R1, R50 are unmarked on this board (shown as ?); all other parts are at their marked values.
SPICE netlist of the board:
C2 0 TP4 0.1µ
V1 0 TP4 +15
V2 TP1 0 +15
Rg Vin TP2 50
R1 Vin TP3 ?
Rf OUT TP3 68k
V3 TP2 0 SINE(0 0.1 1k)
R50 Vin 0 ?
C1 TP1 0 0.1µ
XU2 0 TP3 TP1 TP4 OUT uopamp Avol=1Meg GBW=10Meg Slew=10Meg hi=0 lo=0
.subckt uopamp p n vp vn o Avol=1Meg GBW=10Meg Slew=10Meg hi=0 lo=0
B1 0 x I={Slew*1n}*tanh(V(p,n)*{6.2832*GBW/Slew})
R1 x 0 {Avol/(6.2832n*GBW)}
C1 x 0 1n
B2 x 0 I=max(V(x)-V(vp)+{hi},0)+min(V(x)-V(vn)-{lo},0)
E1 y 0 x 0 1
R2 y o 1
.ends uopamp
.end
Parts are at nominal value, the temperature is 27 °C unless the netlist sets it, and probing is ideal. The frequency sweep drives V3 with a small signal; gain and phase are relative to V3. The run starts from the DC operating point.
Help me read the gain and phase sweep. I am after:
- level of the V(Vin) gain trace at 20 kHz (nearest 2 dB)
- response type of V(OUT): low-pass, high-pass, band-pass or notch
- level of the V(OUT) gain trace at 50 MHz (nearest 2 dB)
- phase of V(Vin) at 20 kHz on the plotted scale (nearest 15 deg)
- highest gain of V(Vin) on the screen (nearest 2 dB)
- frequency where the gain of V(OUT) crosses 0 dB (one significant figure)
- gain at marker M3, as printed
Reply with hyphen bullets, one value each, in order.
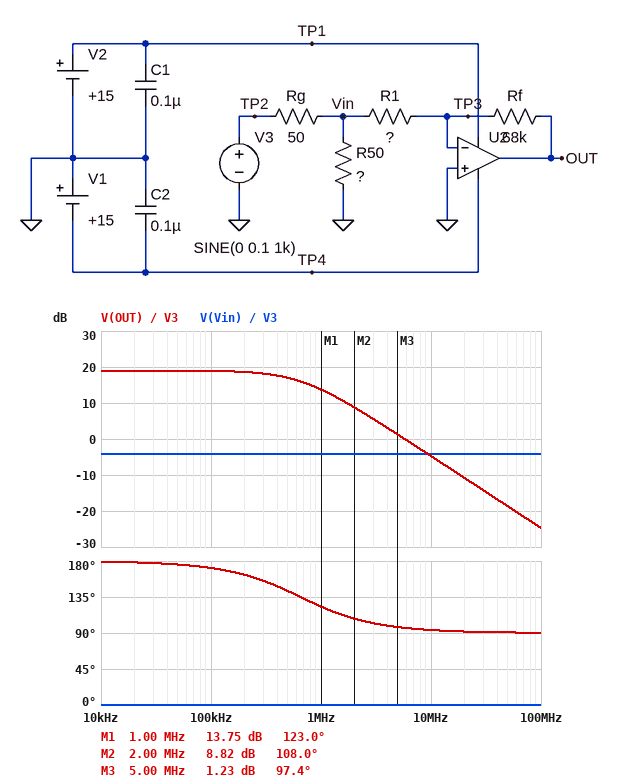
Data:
- -4 dB
- low-pass
- -18 dB
- 0 deg
- -4 dB
- 6 MHz
- 1.23 dB
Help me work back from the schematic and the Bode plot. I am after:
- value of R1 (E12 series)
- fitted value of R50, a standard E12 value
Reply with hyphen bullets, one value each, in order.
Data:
- 4.7 kΩ
- 82 Ω
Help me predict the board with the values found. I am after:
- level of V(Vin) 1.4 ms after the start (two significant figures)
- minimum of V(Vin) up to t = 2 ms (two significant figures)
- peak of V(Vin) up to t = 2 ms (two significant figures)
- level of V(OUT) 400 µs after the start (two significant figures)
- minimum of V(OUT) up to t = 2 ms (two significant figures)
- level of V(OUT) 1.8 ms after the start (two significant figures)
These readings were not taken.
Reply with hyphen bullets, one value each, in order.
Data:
- 36 mV
- -62 mV
- 62 mV
- -530 mV
- -890 mV
- 850 mV
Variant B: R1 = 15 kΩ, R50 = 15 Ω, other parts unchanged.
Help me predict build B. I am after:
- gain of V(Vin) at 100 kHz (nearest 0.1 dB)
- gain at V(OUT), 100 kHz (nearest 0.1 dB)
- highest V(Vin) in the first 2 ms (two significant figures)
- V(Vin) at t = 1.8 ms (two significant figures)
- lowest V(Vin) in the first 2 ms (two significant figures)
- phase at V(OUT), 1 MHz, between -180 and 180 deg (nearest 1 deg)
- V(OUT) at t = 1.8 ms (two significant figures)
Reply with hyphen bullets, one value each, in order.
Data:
- -12.7 dB
- 0.4 dB
- 23 mV
- -22 mV
- -23 mV
- 151 deg
- 99 mV
